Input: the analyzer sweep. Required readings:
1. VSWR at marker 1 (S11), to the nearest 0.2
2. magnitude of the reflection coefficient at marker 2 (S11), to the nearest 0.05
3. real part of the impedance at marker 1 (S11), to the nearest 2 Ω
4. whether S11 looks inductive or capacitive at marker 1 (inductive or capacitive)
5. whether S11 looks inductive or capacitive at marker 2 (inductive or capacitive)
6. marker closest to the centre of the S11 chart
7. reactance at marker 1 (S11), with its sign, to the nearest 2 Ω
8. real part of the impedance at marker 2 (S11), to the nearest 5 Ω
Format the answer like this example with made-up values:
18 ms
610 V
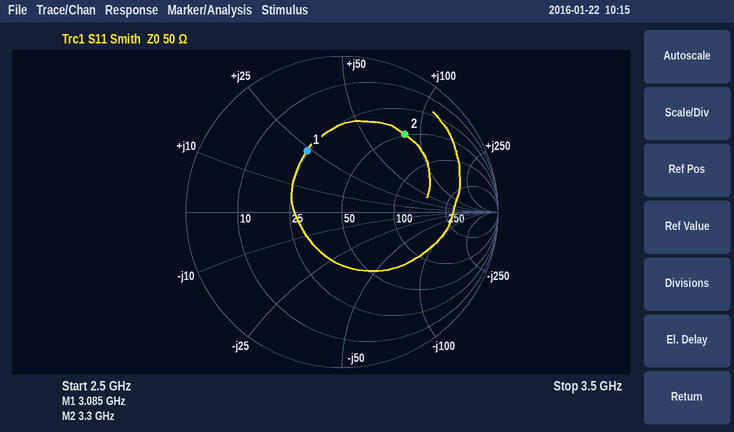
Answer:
2.6
0.65
24 Ω
inductive
inductive
marker 1
+24 Ω
50 Ω
